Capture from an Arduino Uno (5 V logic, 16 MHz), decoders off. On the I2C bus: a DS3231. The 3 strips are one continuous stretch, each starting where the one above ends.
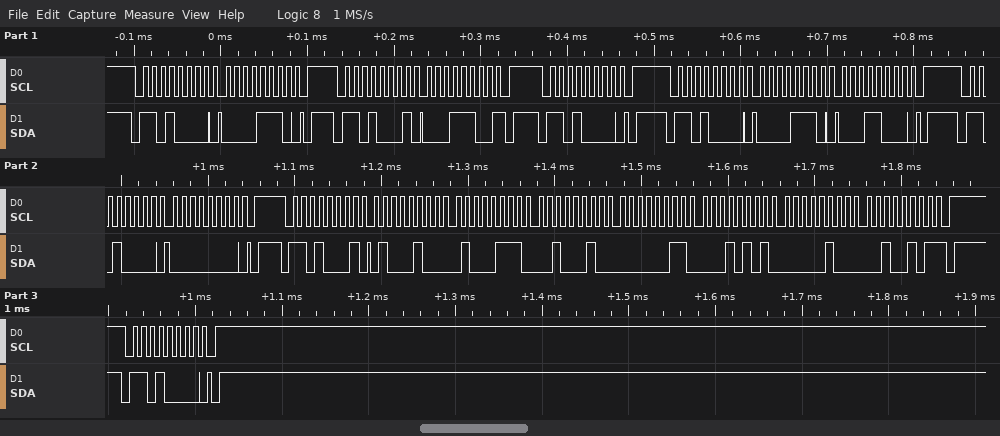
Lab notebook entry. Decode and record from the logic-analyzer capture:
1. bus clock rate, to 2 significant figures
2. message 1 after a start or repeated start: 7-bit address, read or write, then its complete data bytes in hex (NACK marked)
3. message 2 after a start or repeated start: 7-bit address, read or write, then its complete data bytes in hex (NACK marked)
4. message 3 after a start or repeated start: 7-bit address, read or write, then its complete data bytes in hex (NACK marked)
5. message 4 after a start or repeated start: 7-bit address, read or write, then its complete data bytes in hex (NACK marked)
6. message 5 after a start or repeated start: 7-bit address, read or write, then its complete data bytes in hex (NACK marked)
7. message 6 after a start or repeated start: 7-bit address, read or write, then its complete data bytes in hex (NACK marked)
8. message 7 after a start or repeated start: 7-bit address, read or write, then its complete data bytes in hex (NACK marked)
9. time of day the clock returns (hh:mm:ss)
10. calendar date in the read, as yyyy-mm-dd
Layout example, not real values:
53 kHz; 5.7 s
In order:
100 kHz; 0x68 write: 0E; 0x68 read: 1C NACK; 0x68 write; 0x68 write: 0E 18; 0x68 write: 00; 0x68 read: 44 47 22 03 15 04 25 NACK; 0x68 write; 22:47:44; 2025-04-15
